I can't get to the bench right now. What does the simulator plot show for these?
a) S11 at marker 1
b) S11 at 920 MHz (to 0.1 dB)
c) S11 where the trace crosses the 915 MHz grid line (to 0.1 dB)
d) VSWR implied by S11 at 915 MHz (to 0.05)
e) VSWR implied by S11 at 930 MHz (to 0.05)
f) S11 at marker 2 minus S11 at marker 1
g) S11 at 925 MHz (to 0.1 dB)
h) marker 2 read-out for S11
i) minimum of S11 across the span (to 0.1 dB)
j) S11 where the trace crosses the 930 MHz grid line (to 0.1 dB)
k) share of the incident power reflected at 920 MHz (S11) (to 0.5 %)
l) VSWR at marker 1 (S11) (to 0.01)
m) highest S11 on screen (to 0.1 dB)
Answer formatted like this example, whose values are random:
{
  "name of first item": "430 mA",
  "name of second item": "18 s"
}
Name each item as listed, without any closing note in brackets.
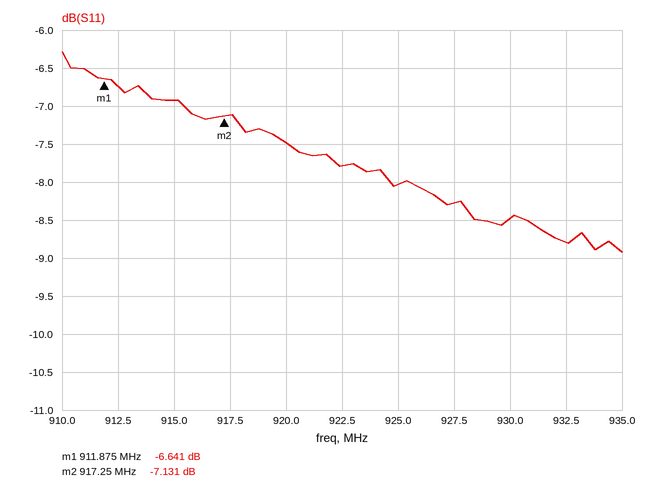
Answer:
{
  "S11 at marker 1": "-6.641 dB",
  "S11 at 920 MHz": "-7.5 dB",
  "S11 where the trace crosses the 915 MHz grid line": "-6.9 dB",
  "VSWR implied by S11 at 915 MHz": "2.65",
  "VSWR implied by S11 at 930 MHz": "2.20",
  "S11 at marker 2 minus S11 at marker 1": "-0.490 dB",
  "S11 at 925 MHz": "-8.0 dB",
  "marker 2 read-out for S11": "-7.131 dB",
  "minimum of S11 across the span": "-8.9 dB",
  "S11 where the trace crosses the 930 MHz grid line": "-8.5 dB",
  "share of the incident power reflected at 920 MHz (S11)": "18.0 %",
  "VSWR at marker 1 (S11)": "2.74",
  "highest S11 on screen": "-6.3 dB"
}
